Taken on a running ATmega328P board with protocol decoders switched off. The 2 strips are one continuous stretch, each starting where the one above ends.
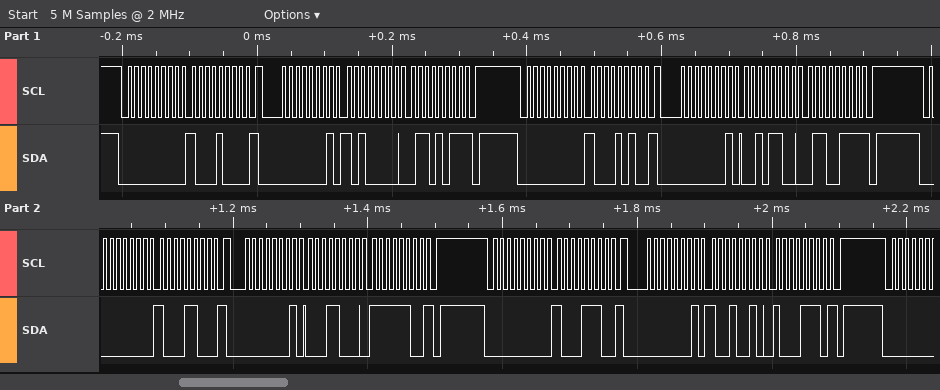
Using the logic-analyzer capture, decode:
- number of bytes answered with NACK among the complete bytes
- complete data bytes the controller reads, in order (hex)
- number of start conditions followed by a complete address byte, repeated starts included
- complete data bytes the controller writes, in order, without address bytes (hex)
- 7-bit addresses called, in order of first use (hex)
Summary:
4
A0 6B 2C 67 18 FC 92 8E
8
88 8A 8C 8E
0x00
